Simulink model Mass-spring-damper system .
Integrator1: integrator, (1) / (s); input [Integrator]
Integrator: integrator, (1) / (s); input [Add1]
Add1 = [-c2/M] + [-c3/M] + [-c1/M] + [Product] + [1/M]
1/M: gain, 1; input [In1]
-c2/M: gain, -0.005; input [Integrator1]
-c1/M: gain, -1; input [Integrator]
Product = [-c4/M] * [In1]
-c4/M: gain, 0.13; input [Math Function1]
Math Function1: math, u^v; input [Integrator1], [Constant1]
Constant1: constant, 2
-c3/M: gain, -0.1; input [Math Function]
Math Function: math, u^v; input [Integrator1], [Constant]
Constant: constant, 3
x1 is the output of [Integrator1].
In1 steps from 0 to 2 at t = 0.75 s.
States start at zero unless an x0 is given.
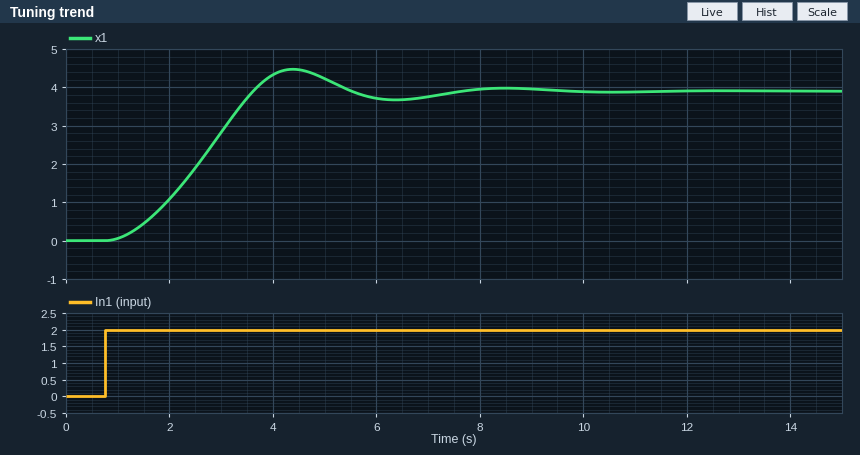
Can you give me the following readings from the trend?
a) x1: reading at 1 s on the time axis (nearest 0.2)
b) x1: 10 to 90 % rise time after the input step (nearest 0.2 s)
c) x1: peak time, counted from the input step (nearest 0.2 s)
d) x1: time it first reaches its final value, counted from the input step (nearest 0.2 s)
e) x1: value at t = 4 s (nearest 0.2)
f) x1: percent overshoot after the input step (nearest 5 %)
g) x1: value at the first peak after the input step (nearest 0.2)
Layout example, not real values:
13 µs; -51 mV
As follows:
0.0; 2.0 s; 3.6 s; 2.8 s; 4.4; 15 %; 4.4
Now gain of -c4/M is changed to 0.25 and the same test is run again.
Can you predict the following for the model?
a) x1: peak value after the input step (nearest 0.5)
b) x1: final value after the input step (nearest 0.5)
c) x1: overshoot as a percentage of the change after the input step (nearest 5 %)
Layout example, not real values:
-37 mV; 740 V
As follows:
6.5; 5.5; 15 %
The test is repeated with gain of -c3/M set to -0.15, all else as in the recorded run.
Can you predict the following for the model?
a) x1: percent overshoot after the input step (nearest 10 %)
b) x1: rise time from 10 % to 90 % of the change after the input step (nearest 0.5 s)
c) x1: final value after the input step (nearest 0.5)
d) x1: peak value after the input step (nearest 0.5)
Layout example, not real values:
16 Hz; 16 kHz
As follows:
20 %; 1.5 s; 3.0; 3.5
